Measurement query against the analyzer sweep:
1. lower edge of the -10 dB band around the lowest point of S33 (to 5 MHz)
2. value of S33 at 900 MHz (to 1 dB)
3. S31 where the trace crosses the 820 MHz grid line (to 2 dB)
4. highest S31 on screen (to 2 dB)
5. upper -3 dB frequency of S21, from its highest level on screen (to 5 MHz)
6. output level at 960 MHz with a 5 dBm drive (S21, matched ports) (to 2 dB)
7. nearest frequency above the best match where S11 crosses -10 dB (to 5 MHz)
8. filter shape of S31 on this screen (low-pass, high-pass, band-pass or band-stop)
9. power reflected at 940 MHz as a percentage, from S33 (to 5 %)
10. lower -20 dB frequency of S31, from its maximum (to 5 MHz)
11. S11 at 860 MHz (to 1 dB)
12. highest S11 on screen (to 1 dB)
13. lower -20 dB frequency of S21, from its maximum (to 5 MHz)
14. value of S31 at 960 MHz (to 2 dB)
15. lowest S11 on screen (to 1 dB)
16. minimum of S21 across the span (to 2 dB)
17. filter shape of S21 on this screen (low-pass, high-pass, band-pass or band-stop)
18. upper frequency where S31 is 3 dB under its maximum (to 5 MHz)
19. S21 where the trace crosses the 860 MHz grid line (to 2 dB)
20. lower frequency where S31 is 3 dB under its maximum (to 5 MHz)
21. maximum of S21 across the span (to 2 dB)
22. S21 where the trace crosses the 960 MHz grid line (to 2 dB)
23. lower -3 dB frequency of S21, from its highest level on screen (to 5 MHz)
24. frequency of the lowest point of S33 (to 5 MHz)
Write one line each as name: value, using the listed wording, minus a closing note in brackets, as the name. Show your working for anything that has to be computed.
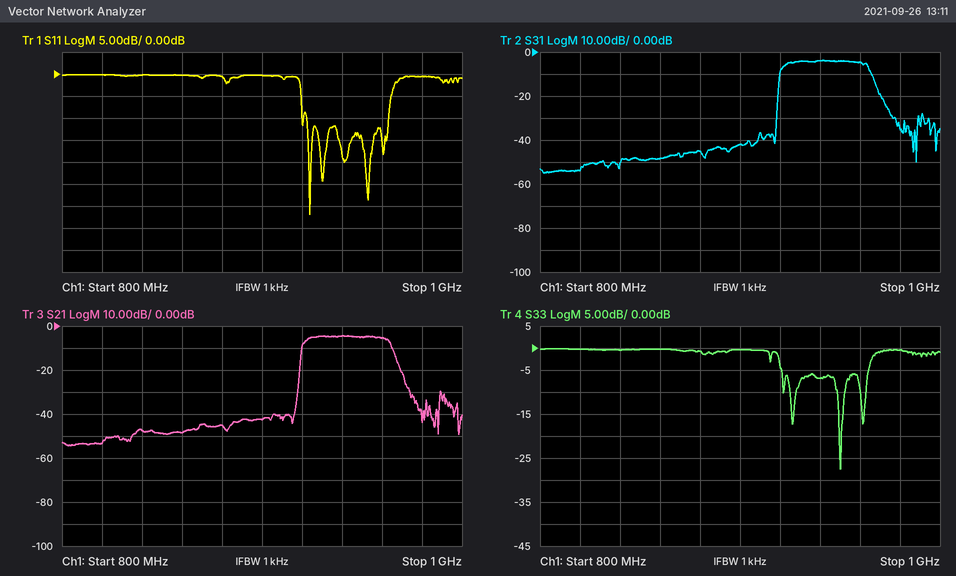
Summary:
lower edge of the -10 dB band around the lowest point of S33: 950 MHz
value of S33 at 900 MHz: 0 dB
S31 where the trace crosses the 820 MHz grid line: -54 dB
highest S31 on screen: -4 dB
upper -3 dB frequency of S21, from its highest level on screen: 965 MHz
output level at 960 MHz with a 5 dBm drive (S21, matched ports): 5 dBm + (-6 dB) = 0 dBm
nearest frequency above the best match where S11 crosses -10 dB: 965 MHz
filter shape of S31 on this screen: band-pass
power reflected at 940 MHz as a percentage, from S33: 10^(-7/10) ≈ 20 %
lower -20 dB frequency of S31, from its maximum: 920 MHz
S11 at 860 MHz: 0 dB
highest S11 on screen: 0 dB
lower -20 dB frequency of S21, from its maximum: 920 MHz
value of S31 at 960 MHz: -4 dB
lowest S11 on screen: -32 dB
minimum of S21 across the span: -54 dB
filter shape of S21 on this screen: band-pass
upper frequency where S31 is 3 dB under its maximum: 965 MHz
S21 where the trace crosses the 860 MHz grid line: -48 dB
lower frequency where S31 is 3 dB under its maximum: 920 MHz
maximum of S21 across the span: -4 dB
S21 where the trace crosses the 960 MHz grid line: -6 dB
lower -3 dB frequency of S21, from its highest level on screen: 920 MHz
frequency of the lowest point of S33: 950 MHz
